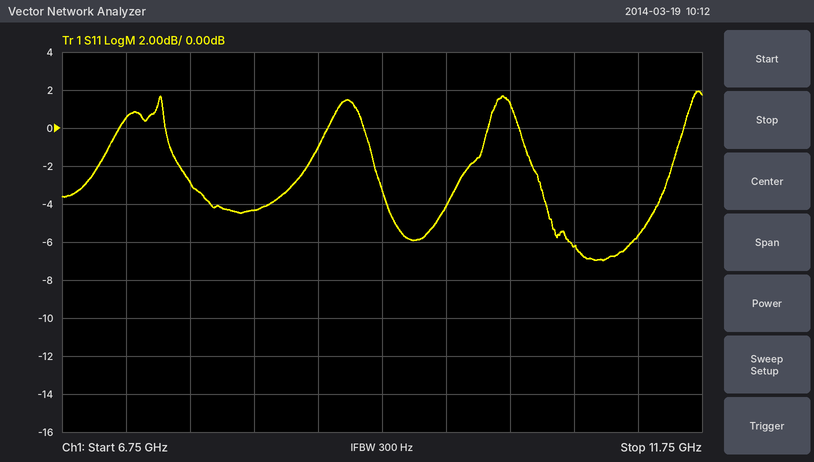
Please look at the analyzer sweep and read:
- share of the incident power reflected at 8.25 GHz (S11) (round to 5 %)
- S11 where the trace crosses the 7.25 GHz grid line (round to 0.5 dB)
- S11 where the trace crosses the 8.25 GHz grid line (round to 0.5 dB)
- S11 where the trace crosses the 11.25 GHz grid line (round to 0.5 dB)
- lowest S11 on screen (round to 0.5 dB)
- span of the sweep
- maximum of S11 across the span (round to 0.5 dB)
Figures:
35 %
0.5 dB
-4.5 dB
-5.5 dB
-7.0 dB
5 GHz
2.0 dB
